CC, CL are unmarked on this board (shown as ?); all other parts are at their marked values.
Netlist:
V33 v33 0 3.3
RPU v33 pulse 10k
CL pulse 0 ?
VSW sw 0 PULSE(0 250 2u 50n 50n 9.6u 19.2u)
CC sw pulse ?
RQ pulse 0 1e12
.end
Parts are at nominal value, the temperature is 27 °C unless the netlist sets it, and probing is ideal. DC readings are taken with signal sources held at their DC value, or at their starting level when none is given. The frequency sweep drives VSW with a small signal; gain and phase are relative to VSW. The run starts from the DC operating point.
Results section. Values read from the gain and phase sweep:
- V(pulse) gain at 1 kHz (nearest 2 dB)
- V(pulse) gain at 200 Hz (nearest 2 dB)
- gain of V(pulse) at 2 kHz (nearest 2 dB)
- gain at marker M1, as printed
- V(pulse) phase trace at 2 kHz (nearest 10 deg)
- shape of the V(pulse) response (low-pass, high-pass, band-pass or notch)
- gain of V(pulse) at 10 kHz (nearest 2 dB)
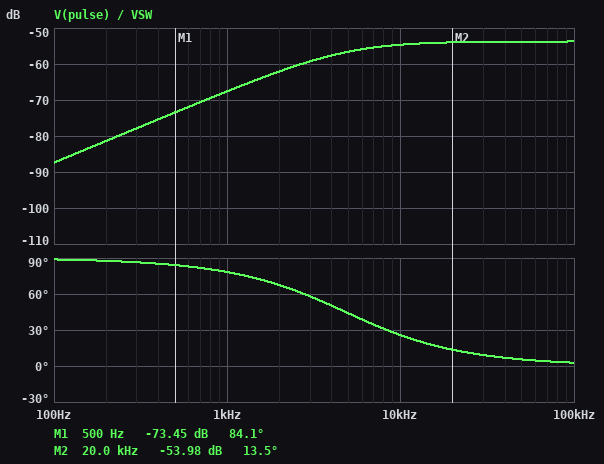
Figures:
-68 dB
-82 dB
-62 dB
-73.45 dB
70 deg
high-pass
-54 dB
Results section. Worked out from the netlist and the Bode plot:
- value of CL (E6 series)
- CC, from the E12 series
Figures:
3.3 nF
6.8 pF
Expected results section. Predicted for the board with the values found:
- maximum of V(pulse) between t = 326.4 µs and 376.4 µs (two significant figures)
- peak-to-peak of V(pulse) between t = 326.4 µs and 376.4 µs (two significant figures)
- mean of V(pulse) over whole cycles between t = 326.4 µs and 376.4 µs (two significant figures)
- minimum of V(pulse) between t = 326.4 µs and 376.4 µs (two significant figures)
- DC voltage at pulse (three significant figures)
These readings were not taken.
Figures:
3.6 V
590 mV
3.3 V
3.0 V
3.30 V
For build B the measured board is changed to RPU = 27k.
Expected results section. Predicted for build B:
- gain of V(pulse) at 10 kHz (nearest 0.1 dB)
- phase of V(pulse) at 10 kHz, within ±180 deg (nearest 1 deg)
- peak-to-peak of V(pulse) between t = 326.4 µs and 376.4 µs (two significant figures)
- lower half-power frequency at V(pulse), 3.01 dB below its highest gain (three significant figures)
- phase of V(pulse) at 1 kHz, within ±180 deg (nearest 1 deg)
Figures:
-53.9 dB
10 deg
540 mV
1.78 kHz
61 deg
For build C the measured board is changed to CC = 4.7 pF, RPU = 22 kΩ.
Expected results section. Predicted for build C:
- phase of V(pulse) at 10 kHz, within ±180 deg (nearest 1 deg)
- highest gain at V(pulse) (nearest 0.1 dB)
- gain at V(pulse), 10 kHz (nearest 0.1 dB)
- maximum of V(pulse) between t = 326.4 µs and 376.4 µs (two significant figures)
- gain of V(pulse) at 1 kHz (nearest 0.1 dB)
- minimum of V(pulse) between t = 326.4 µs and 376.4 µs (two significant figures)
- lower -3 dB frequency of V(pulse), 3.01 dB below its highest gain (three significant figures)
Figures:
12 deg
-56.9 dB
-57.1 dB
3.5 V
-64.6 dB
3.1 V
2.19 kHz
